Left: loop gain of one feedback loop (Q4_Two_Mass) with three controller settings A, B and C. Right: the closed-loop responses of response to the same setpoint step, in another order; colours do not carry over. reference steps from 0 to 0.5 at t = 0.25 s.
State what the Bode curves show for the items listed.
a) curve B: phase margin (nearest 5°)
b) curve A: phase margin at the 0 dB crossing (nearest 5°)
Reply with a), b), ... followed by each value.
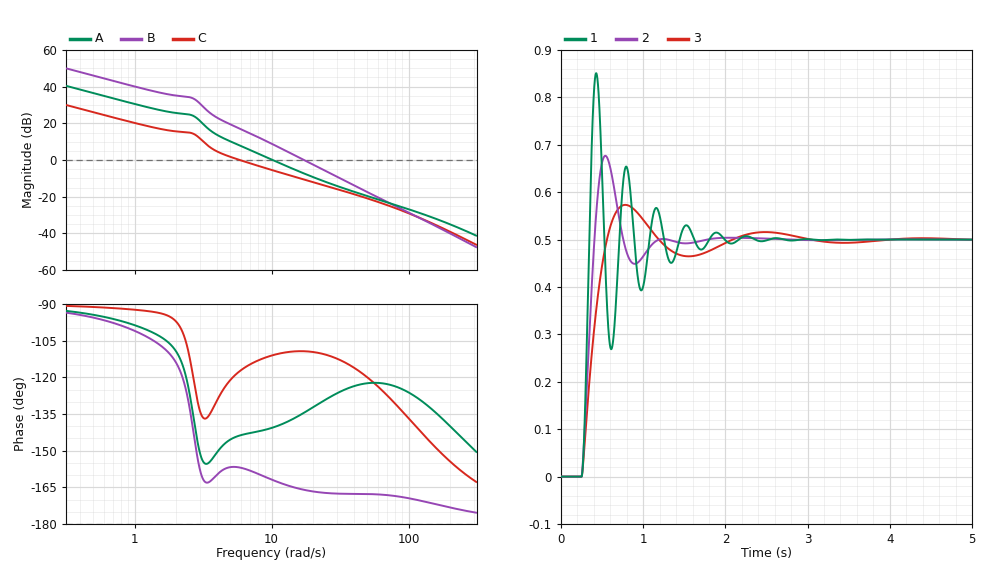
a) 15°
b) 40°
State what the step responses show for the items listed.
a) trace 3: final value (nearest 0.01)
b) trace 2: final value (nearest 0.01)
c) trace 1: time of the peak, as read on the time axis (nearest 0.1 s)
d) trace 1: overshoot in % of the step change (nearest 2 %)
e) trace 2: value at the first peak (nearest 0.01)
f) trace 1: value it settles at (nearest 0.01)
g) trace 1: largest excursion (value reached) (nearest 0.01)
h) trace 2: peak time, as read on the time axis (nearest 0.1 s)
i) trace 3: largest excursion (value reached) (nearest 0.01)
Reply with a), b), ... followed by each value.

a) 0.50
b) 0.50
c) 0.4 s
d) 70 %
e) 0.68
f) 0.50
g) 0.85
h) 0.5 s
i) 0.57
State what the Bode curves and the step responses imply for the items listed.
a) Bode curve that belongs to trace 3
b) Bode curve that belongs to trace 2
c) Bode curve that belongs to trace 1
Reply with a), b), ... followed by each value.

a) C
b) A
c) B
